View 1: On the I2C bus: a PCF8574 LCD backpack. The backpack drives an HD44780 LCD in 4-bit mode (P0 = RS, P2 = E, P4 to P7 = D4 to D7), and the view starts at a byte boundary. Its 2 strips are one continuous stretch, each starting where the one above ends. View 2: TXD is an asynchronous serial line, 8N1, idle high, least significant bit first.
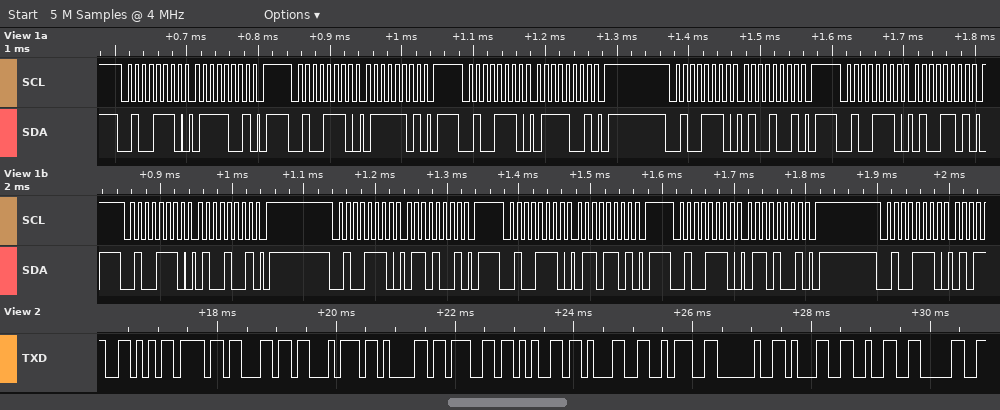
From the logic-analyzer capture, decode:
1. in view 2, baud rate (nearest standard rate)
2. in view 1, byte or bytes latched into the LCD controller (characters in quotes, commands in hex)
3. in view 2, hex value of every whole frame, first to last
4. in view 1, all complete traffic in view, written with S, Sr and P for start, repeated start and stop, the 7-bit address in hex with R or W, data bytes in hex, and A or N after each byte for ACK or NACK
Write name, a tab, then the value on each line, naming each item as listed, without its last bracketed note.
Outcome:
in view 2, baud rate	9600 baud
in view 1, byte or bytes latched into the LCD controller	't'
in view 2, hex value of every whole frame, first to last	0x56 0x6F 0x6C 0x74 0x61 0x67 0x65 0x31 0x3A 0x20 0x31 0x32 0x30
in view 1, all complete traffic in view, written with S, Sr and P for start, repeated start and stop, the 7-bit address in hex with R or W, data bytes in hex, and A or N after each byte for ACK or NACK	S 27W A 79 A P S 27W A 7D A P S 27W A 79 A P S 27W A 49 A P S 27W A 4D A P S 27W A 49 A P S 27W A 69 A P S 27W A 6D A P S 27W A 69 A P S 27W A
